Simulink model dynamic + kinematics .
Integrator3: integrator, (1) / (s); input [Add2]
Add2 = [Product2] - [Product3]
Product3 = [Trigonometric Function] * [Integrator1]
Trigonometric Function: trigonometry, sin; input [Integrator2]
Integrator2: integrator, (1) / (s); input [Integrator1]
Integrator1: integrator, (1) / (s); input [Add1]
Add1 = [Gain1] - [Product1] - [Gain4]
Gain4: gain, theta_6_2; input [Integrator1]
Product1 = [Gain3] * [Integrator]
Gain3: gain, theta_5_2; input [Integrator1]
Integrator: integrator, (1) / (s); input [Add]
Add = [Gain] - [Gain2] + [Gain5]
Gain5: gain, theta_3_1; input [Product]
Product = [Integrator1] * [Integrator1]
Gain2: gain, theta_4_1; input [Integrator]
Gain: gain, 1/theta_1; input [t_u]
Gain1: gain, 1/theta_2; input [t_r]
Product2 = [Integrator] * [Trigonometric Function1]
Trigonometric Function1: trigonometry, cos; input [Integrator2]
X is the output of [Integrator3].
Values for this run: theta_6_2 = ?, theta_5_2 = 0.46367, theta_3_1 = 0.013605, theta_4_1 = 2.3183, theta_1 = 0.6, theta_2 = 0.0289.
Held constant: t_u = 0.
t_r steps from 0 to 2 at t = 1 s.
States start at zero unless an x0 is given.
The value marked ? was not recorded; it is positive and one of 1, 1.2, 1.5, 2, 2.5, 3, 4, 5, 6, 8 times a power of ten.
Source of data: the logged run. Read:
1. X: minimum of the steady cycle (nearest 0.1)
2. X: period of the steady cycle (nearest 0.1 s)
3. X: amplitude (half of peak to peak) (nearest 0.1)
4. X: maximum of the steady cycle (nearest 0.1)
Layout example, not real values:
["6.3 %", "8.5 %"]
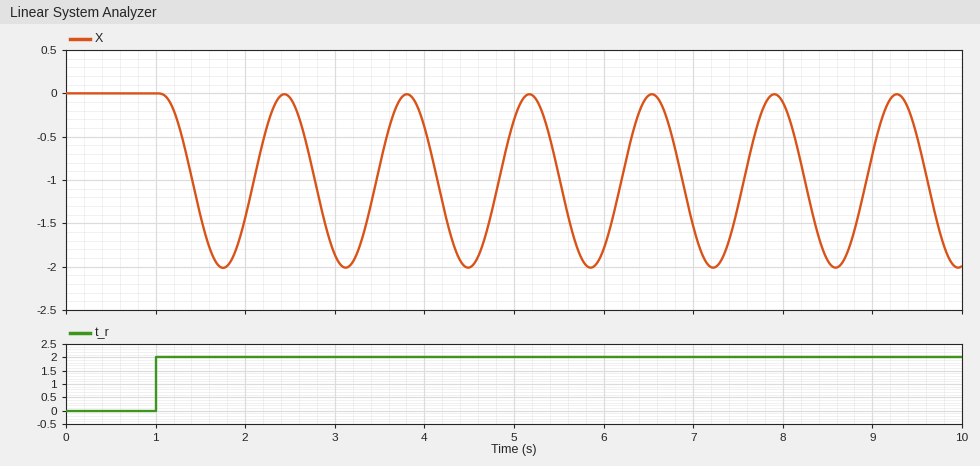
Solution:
["-2.0", "1.4 s", "1.0", "0.0"]
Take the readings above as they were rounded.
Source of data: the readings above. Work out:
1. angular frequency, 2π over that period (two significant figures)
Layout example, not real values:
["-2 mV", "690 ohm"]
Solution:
["4.5 rad/s"]
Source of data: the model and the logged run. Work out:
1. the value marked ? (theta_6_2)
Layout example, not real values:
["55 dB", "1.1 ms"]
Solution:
["15"]
